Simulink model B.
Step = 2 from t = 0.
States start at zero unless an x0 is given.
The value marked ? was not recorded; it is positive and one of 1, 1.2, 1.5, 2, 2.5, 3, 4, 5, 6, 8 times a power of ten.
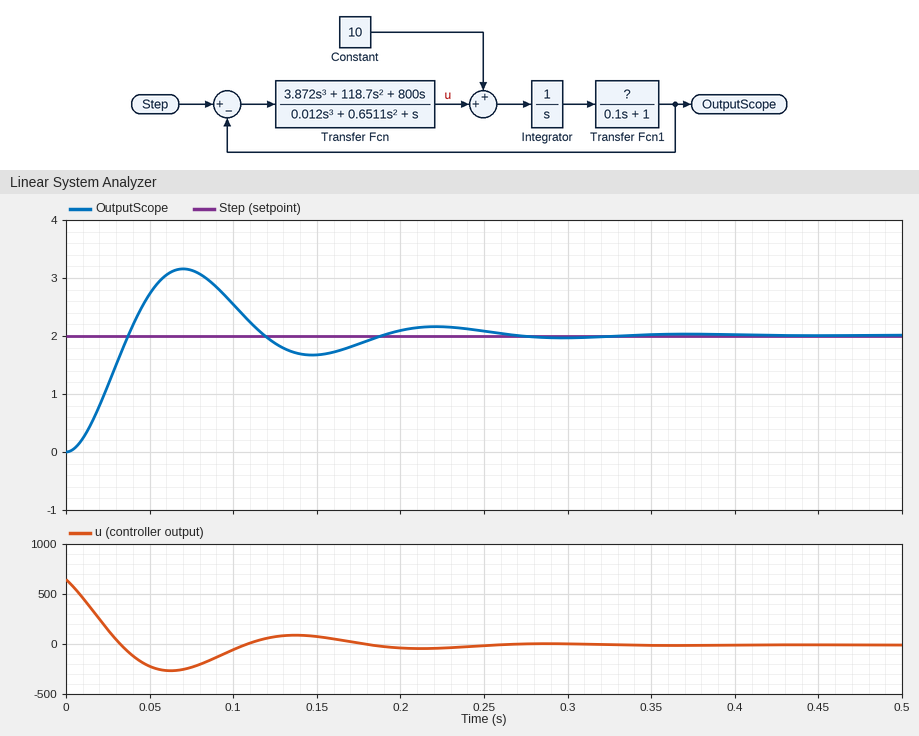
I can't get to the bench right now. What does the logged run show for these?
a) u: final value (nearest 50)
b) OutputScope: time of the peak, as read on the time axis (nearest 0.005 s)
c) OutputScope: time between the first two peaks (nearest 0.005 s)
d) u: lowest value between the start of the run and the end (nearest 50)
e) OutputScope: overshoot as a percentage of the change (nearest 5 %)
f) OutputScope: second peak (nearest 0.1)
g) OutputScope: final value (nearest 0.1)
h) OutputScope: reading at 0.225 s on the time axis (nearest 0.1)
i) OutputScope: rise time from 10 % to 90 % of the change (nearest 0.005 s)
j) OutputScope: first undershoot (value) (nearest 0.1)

0
0.070 s
0.150 s
-250
55 %
2.2
2.0
2.2
0.025 s
1.7
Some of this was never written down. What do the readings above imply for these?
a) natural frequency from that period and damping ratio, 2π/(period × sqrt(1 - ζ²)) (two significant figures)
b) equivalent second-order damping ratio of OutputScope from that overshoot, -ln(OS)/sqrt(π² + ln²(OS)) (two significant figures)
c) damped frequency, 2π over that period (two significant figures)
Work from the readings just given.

43 rad/s
0.19
42 rad/s
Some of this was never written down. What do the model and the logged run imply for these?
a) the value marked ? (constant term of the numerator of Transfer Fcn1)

0.8
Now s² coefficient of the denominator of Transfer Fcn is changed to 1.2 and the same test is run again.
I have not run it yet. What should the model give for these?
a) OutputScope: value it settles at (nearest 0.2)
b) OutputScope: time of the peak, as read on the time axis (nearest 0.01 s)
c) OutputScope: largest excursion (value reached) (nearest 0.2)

2.0
0.10 s
2.8
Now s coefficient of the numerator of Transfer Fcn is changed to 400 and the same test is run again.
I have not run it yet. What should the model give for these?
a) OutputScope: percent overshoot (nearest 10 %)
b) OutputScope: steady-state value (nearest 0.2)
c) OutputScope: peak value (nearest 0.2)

50 %
2.0
3.0
